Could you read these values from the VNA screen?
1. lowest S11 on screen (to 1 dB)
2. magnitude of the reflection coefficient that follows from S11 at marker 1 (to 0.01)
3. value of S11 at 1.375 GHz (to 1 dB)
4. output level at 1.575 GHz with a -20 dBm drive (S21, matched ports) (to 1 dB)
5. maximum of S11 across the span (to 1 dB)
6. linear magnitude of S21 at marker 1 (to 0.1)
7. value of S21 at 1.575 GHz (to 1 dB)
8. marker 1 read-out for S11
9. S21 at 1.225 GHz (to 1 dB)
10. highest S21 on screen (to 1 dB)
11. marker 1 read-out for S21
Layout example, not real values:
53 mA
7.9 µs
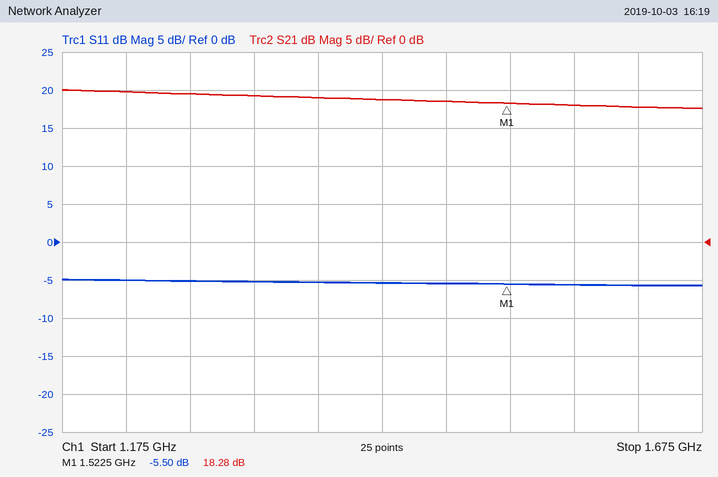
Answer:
-6 dB
0.53
-5 dB
-2 dBm
-5 dB
8.2
18 dB
-5.50 dB
20 dB
20 dB
18.28 dB
